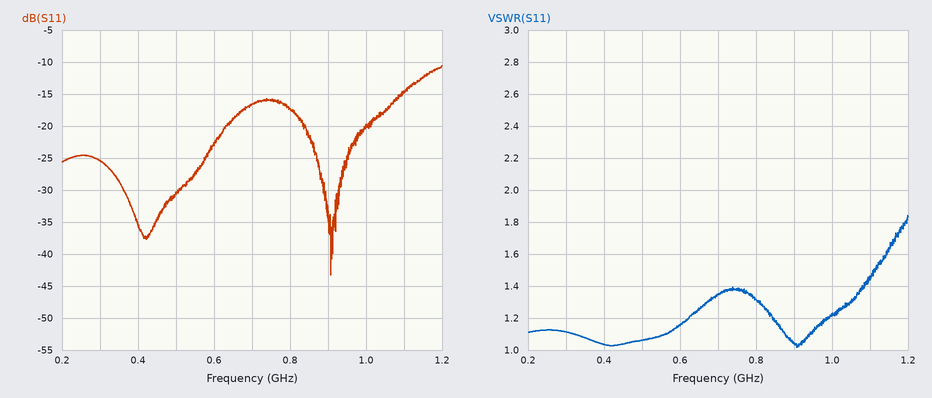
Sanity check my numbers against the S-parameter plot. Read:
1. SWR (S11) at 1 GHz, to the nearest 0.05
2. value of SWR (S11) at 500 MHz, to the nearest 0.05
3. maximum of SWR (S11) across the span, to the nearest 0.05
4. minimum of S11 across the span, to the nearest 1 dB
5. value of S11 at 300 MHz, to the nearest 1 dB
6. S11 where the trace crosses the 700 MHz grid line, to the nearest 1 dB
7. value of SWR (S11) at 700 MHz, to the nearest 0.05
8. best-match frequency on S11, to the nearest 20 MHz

1.20
1.05
1.85
-43 dB
-25 dB
-17 dB
1.35
900 MHz
